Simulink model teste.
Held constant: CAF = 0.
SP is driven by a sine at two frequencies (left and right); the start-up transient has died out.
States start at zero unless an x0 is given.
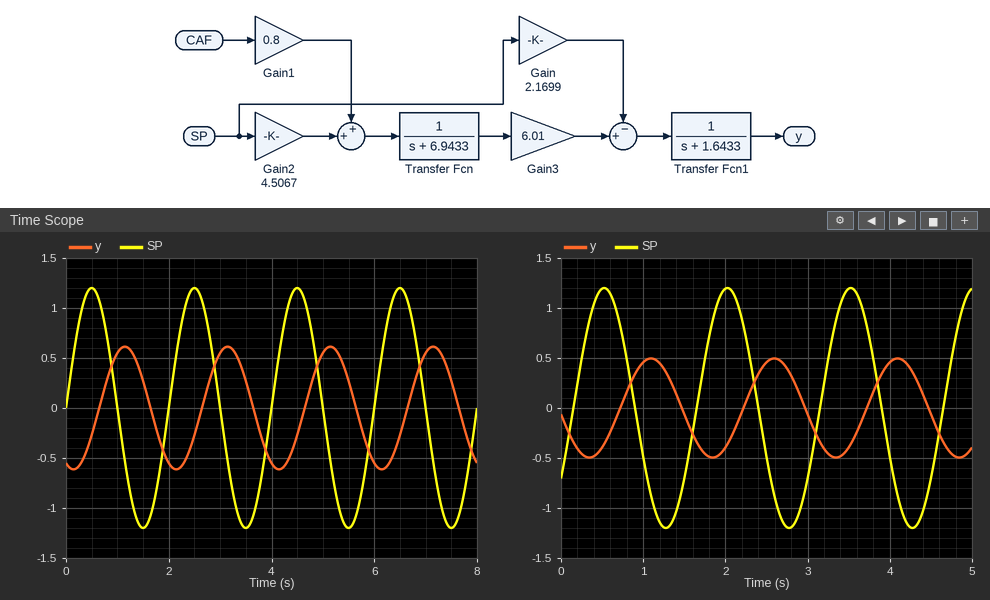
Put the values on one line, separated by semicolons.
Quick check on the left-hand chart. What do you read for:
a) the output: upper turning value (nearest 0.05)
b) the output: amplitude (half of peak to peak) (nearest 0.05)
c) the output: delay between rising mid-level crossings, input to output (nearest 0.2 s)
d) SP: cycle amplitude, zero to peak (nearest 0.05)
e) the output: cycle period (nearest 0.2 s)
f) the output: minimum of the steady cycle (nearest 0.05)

0.60; 0.60; 0.6 s; 1.20; 2.0 s; -0.60
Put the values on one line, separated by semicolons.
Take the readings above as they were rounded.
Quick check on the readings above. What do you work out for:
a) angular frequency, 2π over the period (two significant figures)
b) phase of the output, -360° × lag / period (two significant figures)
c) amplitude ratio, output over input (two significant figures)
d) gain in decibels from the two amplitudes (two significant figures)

3.1 rad/s; -110°; 0.50; -6.0 dB
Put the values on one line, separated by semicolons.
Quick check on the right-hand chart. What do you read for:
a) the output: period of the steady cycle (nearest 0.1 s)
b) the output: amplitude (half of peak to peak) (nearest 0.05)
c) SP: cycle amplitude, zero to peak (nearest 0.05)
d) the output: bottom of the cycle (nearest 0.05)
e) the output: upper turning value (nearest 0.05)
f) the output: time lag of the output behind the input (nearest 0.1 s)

1.5 s; 0.50; 1.20; -0.50; 0.50; 0.6 s
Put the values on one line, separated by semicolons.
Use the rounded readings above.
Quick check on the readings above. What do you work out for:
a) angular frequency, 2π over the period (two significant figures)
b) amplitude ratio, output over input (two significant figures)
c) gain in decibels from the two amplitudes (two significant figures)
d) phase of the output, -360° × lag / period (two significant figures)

4.2 rad/s; 0.42; -7.6 dB; -140°
